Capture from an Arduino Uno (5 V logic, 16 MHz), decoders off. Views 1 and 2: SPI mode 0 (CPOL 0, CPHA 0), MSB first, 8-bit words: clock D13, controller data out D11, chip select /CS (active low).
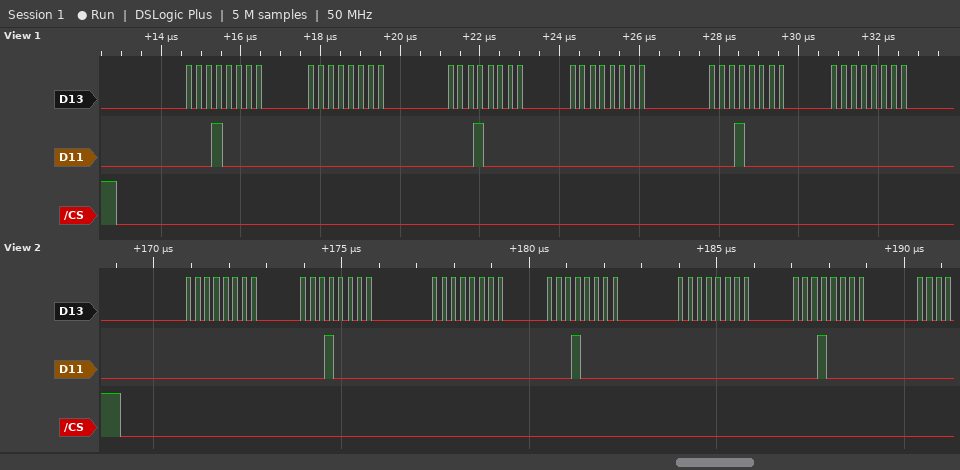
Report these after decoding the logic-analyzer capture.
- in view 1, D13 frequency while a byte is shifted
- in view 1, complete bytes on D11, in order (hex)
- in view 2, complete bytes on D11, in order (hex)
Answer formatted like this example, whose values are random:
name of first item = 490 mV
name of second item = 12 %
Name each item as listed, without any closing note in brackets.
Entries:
in view 1, D13 frequency while a byte is shifted = 4 MHz
in view 1, complete bytes on D11, in order = 10 00 10 00 10 00
in view 2, complete bytes on D11, in order = 00 10 00 10 00 10
